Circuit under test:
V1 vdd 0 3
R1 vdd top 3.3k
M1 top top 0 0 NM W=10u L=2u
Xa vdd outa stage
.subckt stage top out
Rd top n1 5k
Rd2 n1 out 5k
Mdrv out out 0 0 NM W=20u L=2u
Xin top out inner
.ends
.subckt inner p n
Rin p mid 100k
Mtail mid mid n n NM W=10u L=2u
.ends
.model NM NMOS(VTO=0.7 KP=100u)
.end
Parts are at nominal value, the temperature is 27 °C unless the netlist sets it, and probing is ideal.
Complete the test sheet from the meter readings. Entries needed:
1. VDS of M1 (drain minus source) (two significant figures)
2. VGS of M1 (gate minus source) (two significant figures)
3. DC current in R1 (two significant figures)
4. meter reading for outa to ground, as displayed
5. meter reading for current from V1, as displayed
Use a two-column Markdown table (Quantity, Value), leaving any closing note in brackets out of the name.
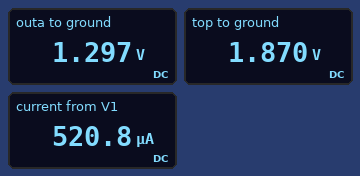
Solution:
| Quantity | Value |
|---|---|
| VDS of M1 (drain minus source) | 1.9 V |
| VGS of M1 (gate minus source) | 1.9 V |
| DC current in R1 | 340 µA |
| meter reading for outa to ground, as displayed | 1.297 V |
| meter reading for current from V1, as displayed | 520.8 µA |
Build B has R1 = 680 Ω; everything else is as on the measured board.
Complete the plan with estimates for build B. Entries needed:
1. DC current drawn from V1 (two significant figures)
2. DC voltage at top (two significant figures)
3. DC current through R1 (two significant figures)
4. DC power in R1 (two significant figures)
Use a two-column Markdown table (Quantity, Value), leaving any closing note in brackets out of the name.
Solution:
| Quantity | Value |
|---|---|
| DC current drawn from V1 | 960 µA |
| DC voltage at top | 2.5 V |
| DC current through R1 | 780 µA |
| DC power in R1 | 420 µW |
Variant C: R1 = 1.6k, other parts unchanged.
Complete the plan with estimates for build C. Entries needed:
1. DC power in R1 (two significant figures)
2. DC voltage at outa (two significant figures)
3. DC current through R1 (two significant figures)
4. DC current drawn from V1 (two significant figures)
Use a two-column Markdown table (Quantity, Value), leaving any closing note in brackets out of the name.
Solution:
| Quantity | Value |
|---|---|
| DC power in R1 | 450 µW |
| DC voltage at outa | 1.3 V |
| DC current through R1 | 530 µA |
| DC current drawn from V1 | 710 µA |
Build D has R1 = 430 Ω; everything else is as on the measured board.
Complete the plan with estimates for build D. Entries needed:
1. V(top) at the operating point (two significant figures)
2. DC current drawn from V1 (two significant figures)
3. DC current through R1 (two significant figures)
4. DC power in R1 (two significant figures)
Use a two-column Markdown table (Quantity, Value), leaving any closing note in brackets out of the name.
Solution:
| Quantity | Value |
|---|---|
| V(top) at the operating point | 2.6 V |
| DC current drawn from V1 | 1.1 mA |
| DC current through R1 | 910 µA |
| DC power in R1 | 360 µW |
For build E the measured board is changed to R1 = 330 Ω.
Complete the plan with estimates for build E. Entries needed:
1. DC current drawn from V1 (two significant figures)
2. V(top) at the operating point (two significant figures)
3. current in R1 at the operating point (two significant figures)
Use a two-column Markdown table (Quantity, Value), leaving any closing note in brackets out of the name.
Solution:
| Quantity | Value |
|---|---|
| DC current drawn from V1 | 1.2 mA |
| V(top) at the operating point | 2.7 V |
| current in R1 at the operating point | 980 µA |
